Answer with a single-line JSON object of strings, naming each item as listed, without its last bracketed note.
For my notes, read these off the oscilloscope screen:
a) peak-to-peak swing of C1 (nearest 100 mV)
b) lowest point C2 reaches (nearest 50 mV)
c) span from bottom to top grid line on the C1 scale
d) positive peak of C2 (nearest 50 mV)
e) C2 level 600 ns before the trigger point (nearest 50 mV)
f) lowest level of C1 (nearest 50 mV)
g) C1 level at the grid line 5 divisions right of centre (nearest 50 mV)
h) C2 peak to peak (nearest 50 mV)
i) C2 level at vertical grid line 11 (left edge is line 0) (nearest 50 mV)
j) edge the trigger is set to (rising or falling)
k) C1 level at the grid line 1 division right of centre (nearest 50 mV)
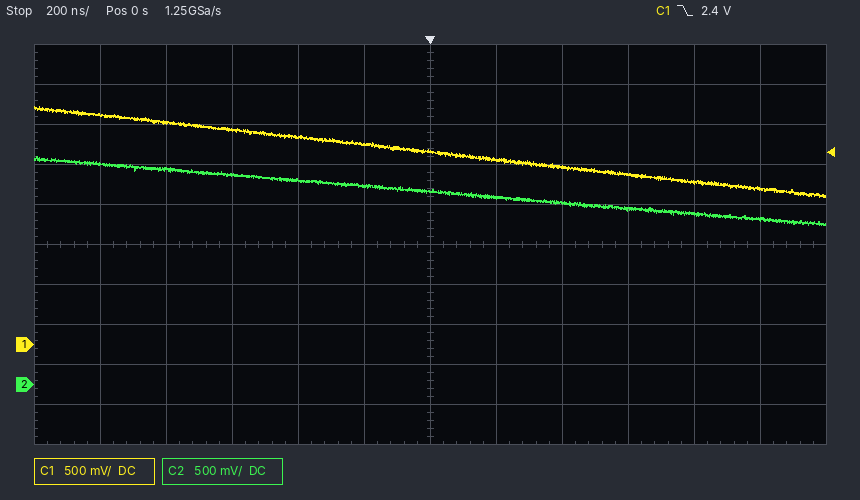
{"peak-to-peak swing of C1": "1.10 V", "lowest point C2 reaches": "2.00 V", "span from bottom to top grid line on the C1 scale": "5 V", "positive peak of C2": "2.85 V", "C2 level 600 ns before the trigger point": "2.60 V", "lowest level of C1": "1.85 V", "C1 level at the grid line 5 divisions right of centre": "1.95 V", "C2 peak to peak": "850 mV", "C2 level at vertical grid line 11 (left edge is line 0)": "2.05 V", "edge the trigger is set to": "falling", "C1 level at the grid line 1 division right of centre": "2.30 V"}
